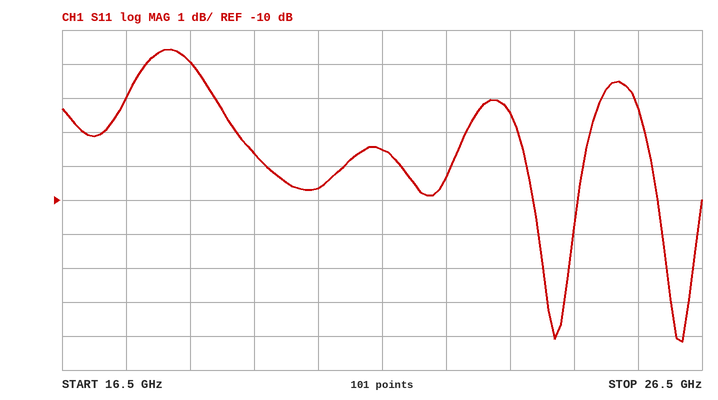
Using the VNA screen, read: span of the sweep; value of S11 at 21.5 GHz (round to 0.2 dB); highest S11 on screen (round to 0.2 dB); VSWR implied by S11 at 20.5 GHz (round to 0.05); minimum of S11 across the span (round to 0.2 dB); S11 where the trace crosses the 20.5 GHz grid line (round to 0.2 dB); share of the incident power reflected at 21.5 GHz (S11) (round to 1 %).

10 GHz
-8.6 dB
-5.6 dB
2.00
-14.2 dB
-9.6 dB
14 %
